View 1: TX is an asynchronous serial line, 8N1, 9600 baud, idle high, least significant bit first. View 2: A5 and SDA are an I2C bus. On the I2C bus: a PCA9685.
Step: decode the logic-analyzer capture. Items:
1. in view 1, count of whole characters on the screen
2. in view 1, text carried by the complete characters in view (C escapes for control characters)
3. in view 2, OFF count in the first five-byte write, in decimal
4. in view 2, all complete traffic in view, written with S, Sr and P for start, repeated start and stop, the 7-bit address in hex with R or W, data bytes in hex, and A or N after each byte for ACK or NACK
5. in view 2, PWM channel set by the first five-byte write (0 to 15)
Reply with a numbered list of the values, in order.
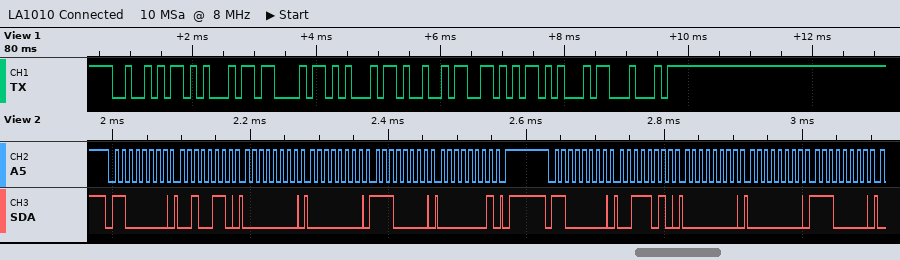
1. 8
2. "RECEIVED"
3. 480
4. S 60W A 26 A 00 A 00 A E0 A 01 A P S 60W A 3A A 00 A 00 A E0 A
5. 8
